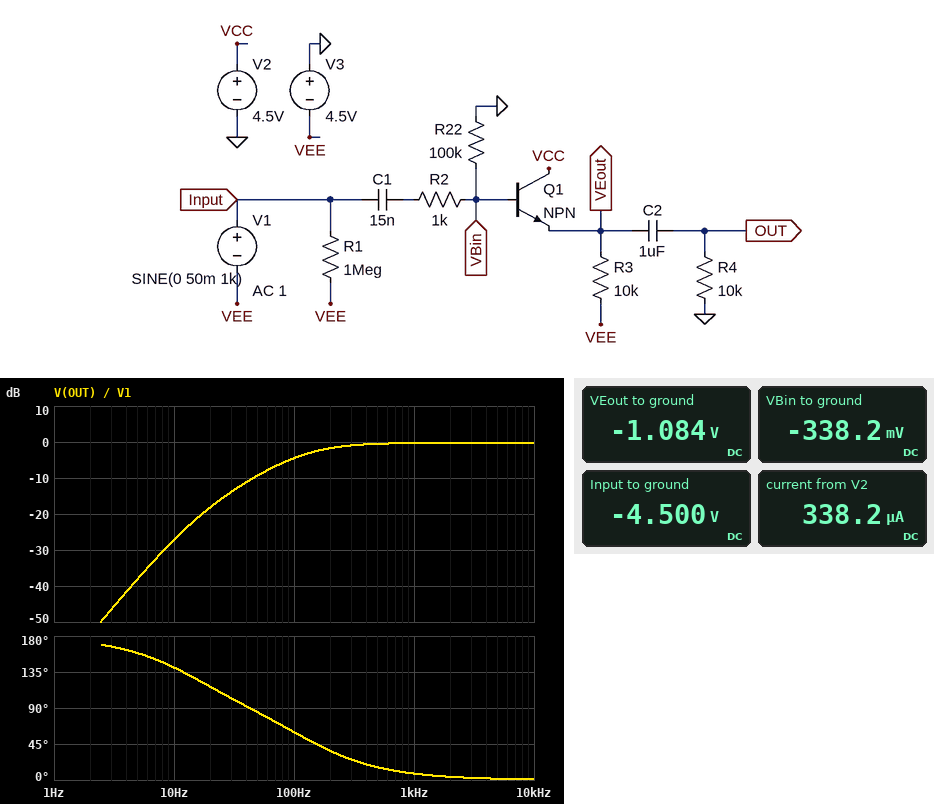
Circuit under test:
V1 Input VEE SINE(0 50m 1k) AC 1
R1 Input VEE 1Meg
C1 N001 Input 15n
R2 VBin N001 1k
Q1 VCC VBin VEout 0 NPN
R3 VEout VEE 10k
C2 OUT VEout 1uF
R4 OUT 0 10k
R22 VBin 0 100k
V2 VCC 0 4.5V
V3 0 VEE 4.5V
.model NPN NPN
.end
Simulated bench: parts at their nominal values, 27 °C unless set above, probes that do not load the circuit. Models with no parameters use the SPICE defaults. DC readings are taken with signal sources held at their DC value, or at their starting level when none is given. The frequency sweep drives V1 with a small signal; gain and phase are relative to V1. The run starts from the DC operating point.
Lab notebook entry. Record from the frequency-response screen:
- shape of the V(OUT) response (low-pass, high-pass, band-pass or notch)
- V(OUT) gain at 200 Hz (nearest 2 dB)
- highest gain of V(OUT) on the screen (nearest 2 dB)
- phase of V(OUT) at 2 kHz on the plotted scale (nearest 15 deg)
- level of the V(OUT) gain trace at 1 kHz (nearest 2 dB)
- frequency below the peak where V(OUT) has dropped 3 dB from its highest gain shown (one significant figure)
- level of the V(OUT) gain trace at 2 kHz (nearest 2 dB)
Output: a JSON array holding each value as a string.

["high-pass", "-2 dB", "0 dB", "0 deg", "0 dB", "100 Hz", "0 dB"]
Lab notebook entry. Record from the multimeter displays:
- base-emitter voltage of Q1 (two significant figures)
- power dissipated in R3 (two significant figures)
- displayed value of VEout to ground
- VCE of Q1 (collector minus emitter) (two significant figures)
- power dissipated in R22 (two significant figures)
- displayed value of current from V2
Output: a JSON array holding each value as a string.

["750 mV", "1.2 mW", "-1.084 V", "5.6 V", "1.1 µW", "338.2 µA"]
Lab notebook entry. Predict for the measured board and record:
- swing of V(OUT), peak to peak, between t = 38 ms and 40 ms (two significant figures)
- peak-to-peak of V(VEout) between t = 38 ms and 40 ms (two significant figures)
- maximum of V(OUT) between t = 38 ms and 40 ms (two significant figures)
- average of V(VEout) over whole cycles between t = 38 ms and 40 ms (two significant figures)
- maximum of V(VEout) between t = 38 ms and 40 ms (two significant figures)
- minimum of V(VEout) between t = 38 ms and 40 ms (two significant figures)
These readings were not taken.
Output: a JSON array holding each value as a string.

["97 mV", "97 mV", "48 mV", "-1.1 V", "-1.0 V", "-1.1 V"]
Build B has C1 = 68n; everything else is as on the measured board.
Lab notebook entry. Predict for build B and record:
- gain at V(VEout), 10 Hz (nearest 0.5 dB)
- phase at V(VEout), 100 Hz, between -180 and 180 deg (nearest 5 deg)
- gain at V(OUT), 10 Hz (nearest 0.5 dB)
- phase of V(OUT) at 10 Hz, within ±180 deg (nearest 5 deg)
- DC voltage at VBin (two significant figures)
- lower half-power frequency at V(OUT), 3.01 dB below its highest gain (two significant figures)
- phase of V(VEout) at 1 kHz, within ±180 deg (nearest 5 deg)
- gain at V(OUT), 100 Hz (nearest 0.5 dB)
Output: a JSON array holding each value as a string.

["-9.0 dB", "15 deg", "-14.5 dB", "125 deg", "-340 mV", "35 Hz", "0 deg", "-0.5 dB"]
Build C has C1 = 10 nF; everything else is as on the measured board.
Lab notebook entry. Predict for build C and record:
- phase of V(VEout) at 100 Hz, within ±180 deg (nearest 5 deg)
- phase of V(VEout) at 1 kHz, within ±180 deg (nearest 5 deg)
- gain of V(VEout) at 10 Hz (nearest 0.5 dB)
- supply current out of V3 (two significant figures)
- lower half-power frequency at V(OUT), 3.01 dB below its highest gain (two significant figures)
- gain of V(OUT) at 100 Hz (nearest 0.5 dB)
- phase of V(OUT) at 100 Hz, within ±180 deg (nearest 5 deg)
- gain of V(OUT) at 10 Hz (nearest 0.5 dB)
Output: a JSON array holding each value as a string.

["60 deg", "10 deg", "-25.0 dB", "340 µA", "190 Hz", "-7.0 dB", "70 deg", "-30.5 dB"]
